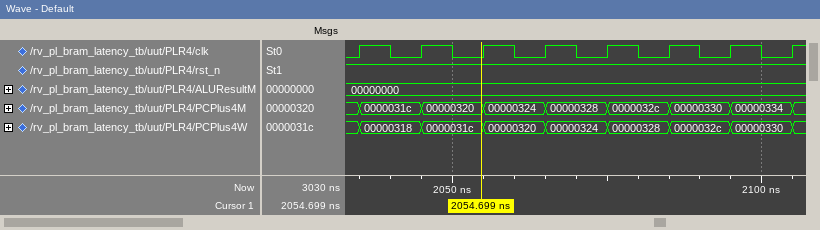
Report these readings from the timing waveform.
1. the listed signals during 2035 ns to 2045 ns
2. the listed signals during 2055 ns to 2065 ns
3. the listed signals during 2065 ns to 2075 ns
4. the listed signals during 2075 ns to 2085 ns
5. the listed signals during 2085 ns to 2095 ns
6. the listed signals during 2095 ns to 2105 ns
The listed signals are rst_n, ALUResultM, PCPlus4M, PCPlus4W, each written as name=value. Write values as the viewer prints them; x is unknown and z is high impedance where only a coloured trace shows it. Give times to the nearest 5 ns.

rst_n=1, ALUResultM=00000000, PCPlus4M=0000031c, PCPlus4W=00000318
rst_n=1, ALUResultM=00000000, PCPlus4M=00000324, PCPlus4W=00000320
rst_n=1, ALUResultM=00000000, PCPlus4M=00000328, PCPlus4W=00000324
rst_n=1, ALUResultM=00000000, PCPlus4M=0000032c, PCPlus4W=00000328
rst_n=1, ALUResultM=00000000, PCPlus4M=00000330, PCPlus4W=0000032c
rst_n=1, ALUResultM=00000000, PCPlus4M=00000334, PCPlus4W=00000330
